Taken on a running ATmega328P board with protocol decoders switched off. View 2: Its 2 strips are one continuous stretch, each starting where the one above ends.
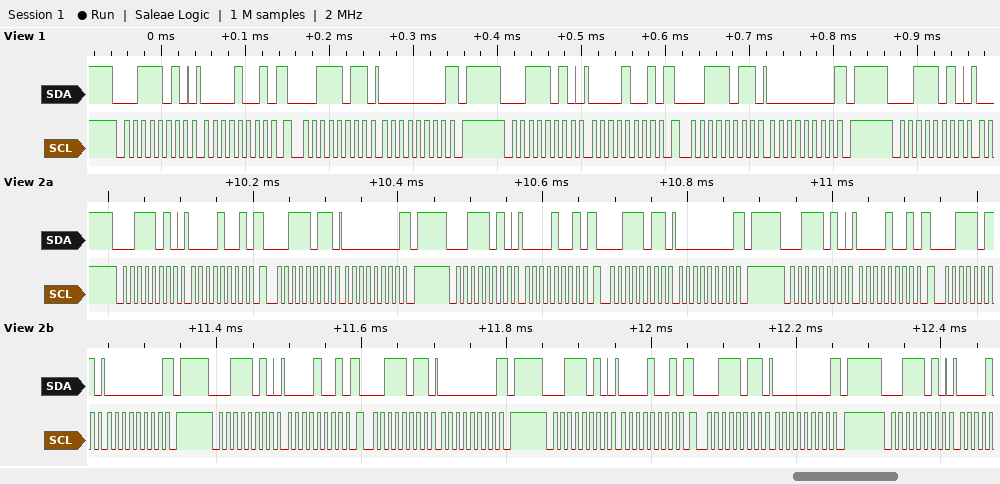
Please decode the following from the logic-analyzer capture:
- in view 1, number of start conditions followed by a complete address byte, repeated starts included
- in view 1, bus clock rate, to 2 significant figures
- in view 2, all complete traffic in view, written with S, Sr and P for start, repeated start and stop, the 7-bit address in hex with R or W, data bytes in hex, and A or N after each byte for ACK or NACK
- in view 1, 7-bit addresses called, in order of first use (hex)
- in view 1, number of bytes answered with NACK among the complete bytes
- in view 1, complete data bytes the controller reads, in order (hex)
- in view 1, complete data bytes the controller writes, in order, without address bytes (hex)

5
100 kHz
S 1DW A 09 A Sr 1DR A 00 N P S 1DW A 09 A Sr 1DR A 00 N P S 1DW A 09 A Sr 1DR A 00 N P S 1DW A 09 A Sr 1DR A 00 N P S 1DW A 09 A Sr 1DR A 00 N P S 1DW A
0x1D
2
00 00
09 09
